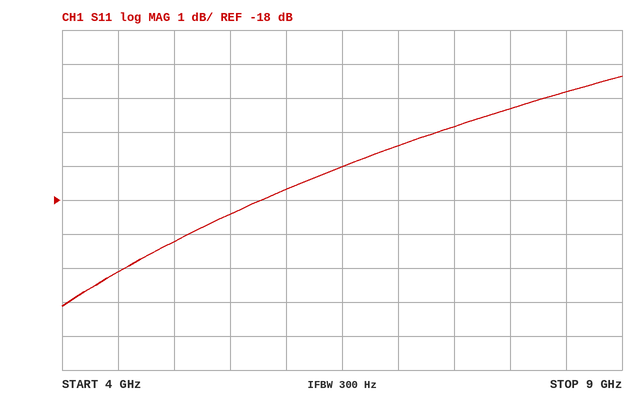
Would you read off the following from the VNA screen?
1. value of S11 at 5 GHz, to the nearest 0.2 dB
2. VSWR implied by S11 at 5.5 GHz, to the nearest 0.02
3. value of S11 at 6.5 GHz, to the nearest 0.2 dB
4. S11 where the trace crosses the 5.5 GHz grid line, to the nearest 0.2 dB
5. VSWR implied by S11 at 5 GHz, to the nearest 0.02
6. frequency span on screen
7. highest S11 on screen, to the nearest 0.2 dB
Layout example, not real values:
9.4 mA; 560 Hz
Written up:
-19.2 dB; 1.28; -17.0 dB; -18.4 dB; 1.24; 5 GHz; -14.4 dB
